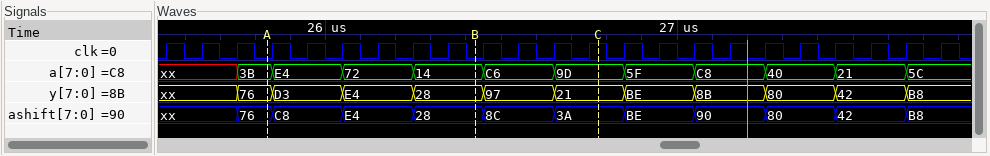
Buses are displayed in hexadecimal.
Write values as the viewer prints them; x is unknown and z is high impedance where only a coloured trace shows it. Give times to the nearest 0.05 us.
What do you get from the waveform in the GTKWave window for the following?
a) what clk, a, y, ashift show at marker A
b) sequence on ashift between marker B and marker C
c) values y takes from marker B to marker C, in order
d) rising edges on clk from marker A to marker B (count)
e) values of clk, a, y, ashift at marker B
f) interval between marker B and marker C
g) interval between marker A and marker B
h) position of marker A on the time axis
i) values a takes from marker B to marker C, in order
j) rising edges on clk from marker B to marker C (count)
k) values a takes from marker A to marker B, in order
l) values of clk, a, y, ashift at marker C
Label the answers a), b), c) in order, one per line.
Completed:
a) clk=0, a=3B, y=76, ashift=76
b) 28, 8C, 3A
c) 28, 97, 21
d) 6
e) clk=0, a=14, y=28, ashift=28
f) 0.35 us
g) 0.6 us
h) 25.85 us
i) 14, C6, 9D
j) 4
k) 3B, E4, 72, 14
l) clk=1, a=9D, y=21, ashift=3A
